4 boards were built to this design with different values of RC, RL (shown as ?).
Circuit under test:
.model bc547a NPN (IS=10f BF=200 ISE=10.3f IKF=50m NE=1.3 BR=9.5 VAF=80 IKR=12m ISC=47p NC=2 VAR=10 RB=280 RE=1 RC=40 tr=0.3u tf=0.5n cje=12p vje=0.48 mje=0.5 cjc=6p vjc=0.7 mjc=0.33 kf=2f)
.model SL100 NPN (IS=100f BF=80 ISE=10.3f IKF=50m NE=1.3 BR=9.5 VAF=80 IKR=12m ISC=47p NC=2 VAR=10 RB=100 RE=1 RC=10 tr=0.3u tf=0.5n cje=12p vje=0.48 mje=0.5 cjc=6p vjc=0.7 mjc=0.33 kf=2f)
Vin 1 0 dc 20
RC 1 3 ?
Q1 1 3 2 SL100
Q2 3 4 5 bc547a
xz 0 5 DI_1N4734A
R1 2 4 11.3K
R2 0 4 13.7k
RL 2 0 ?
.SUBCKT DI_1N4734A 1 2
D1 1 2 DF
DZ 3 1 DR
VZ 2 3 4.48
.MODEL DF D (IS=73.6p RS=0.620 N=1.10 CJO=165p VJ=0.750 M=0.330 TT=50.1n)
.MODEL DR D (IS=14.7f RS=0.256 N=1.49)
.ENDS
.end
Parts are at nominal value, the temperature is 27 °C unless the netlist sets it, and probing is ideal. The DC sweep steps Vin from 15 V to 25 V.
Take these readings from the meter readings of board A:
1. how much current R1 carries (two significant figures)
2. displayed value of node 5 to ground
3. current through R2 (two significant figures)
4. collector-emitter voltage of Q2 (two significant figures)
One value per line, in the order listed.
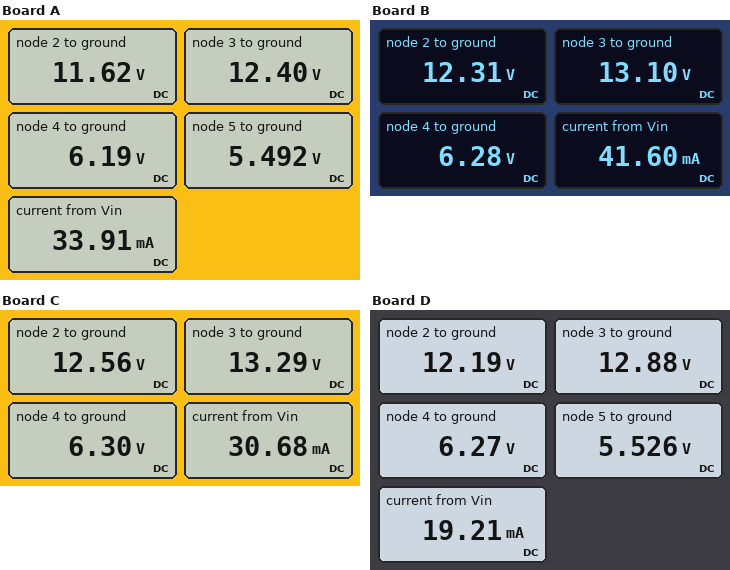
480 µA
5.492 V
450 µA
6.9 V
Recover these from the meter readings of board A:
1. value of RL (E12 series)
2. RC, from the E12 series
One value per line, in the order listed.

390 Ω
1.8 kΩ
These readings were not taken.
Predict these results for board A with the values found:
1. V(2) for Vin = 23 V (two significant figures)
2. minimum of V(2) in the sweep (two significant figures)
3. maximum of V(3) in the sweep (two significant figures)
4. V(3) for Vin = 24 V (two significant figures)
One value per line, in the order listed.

12 V
11 V
13 V
13 V
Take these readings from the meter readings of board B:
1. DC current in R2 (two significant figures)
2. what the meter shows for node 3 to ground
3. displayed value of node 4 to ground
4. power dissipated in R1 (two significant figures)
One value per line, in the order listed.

460 µA
13.10 V
6.28 V
3.2 mW
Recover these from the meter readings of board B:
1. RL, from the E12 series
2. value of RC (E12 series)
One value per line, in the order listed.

390 Ω
680 Ω
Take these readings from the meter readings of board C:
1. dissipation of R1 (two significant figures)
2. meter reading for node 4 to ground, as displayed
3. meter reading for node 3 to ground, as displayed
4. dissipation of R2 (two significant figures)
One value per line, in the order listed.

3.5 mW
6.30 V
13.29 V
2.9 mW
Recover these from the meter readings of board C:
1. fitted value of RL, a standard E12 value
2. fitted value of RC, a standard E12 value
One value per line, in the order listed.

680 Ω
560 Ω
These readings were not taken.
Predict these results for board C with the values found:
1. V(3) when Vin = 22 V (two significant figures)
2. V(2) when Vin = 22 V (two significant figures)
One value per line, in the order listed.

14 V
13 V
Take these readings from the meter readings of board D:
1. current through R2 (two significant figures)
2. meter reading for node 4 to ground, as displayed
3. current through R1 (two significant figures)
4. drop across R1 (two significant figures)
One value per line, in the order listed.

460 µA
6.27 V
520 µA
5.9 V
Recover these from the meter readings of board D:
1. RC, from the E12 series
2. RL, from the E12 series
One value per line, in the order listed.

820 Ω
1.2 kΩ
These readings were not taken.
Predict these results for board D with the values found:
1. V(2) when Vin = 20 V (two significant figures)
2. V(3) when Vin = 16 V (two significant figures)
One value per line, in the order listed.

12 V
12 V
